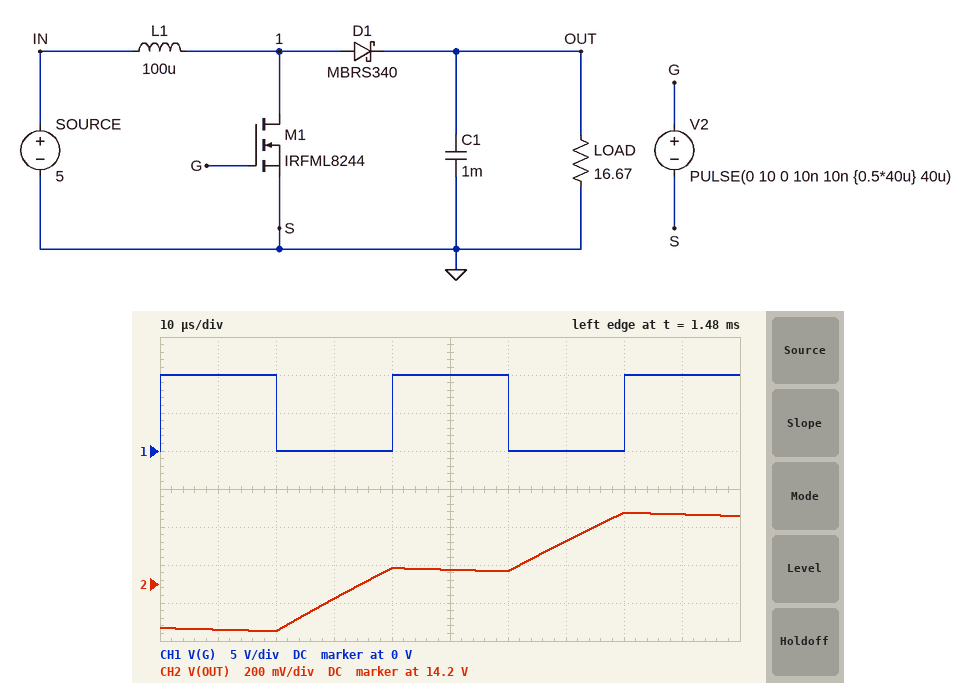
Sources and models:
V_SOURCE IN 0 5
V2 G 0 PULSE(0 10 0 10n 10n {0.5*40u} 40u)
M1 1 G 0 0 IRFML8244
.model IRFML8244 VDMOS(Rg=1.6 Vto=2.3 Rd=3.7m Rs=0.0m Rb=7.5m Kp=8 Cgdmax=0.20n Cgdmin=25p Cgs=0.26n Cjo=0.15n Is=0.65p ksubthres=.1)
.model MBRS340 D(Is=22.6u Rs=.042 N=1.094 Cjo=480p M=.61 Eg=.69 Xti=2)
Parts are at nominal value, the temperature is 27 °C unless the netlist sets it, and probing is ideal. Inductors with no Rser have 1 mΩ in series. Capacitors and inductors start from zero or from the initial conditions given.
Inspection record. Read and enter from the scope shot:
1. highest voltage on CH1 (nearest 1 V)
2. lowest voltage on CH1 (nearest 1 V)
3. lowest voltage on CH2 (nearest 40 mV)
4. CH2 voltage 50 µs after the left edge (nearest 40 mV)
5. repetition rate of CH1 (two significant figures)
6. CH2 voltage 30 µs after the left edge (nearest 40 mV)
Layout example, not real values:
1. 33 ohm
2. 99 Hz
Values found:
1. 10 V
2. 0 V
3. 13.96 V
4. 14.28 V
5. 25 kHz
6. 14.12 V
